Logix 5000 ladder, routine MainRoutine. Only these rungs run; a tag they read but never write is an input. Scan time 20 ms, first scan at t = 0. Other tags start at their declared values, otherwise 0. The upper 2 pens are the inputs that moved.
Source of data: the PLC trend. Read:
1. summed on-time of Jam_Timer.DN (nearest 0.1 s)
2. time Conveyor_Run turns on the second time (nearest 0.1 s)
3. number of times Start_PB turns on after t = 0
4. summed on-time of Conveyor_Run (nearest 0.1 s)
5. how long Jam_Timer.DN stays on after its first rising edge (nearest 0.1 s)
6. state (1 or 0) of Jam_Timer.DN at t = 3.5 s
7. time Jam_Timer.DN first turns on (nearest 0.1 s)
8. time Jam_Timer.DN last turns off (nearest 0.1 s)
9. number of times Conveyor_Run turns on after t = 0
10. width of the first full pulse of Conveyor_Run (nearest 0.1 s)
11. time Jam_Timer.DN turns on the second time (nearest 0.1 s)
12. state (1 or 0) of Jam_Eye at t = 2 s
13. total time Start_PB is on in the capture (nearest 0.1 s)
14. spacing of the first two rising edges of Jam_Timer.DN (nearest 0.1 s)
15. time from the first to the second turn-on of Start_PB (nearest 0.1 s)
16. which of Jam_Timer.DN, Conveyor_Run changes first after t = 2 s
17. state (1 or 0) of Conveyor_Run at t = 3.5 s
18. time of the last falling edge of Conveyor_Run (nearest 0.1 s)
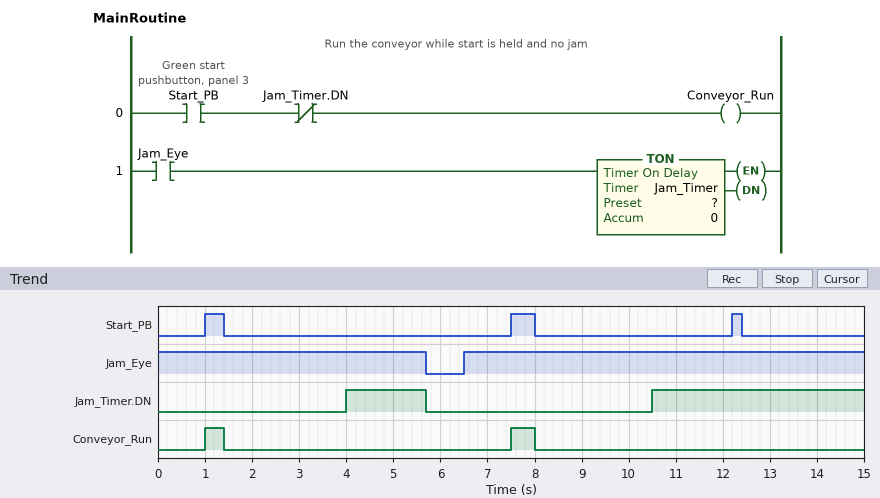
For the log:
6.2 s
7.5 s
3
0.9 s
1.7 s
0
4.0 s
5.7 s
2
0.4 s
10.5 s
1
1.1 s
6.5 s
6.5 s
Jam_Timer.DN
0
8.0 s
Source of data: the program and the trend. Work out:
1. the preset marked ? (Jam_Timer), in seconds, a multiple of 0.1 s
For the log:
4.0 s
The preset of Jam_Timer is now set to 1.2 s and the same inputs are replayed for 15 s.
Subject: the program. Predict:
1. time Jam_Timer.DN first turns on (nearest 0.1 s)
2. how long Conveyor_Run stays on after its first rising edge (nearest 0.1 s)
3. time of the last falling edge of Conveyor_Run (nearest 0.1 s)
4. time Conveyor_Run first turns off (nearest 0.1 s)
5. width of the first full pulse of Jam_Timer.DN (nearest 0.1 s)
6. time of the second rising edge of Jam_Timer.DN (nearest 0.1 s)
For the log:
1.2 s
0.2 s
7.7 s
1.2 s
4.5 s
7.7 s
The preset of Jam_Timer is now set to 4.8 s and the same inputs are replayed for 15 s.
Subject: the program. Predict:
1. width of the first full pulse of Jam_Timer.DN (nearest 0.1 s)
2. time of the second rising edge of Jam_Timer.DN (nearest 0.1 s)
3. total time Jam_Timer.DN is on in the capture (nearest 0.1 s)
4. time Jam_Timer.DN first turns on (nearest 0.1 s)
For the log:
0.9 s
11.3 s
4.6 s
4.8 s
